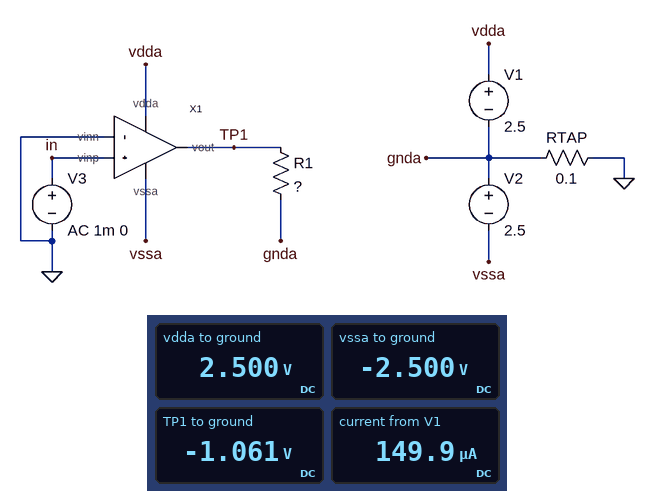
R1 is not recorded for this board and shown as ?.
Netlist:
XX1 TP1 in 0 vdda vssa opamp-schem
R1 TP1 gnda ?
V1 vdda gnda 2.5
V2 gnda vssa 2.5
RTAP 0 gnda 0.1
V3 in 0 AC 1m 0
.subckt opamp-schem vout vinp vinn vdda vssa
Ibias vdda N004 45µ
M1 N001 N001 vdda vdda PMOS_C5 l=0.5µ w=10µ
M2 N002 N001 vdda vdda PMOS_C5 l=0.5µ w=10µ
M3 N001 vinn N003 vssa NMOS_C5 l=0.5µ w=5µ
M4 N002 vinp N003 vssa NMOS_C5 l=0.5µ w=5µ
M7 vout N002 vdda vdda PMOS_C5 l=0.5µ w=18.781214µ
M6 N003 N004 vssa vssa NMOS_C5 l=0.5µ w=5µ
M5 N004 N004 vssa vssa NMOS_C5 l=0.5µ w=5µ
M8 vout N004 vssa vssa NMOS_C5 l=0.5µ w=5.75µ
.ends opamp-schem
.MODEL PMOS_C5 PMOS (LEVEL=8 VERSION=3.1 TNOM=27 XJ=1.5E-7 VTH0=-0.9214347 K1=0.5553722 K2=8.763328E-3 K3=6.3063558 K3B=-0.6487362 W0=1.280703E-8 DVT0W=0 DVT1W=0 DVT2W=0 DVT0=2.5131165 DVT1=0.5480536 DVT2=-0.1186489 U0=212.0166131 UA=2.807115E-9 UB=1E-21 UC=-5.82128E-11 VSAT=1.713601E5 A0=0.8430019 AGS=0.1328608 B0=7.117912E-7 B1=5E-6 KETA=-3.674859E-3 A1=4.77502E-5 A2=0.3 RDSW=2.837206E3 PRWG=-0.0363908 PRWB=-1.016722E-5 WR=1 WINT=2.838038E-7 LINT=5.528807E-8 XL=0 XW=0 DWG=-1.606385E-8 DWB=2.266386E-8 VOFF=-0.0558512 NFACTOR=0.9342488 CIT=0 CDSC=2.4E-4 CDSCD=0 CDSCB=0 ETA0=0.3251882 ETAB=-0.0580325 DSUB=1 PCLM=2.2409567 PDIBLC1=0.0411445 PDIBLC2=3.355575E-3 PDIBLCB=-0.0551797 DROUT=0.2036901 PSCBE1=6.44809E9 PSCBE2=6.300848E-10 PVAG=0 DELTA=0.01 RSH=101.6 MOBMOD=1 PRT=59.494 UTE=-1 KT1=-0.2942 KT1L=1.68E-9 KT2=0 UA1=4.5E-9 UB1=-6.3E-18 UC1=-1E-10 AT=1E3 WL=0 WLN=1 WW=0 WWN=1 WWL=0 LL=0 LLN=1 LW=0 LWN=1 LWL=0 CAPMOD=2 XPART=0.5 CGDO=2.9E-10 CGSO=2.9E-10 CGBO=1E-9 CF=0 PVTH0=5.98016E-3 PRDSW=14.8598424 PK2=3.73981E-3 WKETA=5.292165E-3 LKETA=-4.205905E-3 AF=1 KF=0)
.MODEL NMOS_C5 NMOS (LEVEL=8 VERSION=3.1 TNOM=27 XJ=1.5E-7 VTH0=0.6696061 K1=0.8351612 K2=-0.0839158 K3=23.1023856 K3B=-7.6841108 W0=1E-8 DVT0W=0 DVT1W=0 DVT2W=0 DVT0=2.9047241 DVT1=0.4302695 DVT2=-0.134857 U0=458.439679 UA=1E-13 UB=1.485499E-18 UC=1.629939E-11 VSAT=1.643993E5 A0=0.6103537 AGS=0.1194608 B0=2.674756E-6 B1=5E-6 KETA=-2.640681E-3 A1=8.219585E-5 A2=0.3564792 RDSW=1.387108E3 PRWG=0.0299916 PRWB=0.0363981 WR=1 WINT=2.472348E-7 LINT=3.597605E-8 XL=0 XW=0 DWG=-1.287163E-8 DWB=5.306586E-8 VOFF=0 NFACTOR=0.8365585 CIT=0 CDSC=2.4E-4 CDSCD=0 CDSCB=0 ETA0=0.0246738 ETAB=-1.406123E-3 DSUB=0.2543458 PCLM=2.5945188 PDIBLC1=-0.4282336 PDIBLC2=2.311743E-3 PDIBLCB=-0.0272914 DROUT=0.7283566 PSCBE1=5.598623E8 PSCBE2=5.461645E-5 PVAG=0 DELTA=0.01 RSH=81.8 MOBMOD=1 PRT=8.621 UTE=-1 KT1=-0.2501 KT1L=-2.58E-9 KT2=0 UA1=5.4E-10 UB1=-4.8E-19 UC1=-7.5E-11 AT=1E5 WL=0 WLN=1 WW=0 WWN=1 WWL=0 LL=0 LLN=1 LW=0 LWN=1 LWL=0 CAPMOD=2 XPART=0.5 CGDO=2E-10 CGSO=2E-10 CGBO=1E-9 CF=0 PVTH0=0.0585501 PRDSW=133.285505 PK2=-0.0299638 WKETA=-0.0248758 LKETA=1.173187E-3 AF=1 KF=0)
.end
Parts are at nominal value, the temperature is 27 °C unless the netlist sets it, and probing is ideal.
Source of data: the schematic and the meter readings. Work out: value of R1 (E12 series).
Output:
390 kΩ
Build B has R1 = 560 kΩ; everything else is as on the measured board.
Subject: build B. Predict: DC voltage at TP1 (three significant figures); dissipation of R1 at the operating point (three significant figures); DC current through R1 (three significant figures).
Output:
-1.12 V
2.23 µW
1.99 µA
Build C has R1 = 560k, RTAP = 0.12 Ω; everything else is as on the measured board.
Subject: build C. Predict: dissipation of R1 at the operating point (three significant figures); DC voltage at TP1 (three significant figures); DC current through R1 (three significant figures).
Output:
2.23 µW
-1.12 V
1.99 µA
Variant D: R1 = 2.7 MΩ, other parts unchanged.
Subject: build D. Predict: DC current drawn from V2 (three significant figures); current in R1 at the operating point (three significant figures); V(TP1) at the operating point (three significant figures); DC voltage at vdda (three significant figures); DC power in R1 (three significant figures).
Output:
151 µA
456 nA
-1.23 V
2.50 V
562 nW
